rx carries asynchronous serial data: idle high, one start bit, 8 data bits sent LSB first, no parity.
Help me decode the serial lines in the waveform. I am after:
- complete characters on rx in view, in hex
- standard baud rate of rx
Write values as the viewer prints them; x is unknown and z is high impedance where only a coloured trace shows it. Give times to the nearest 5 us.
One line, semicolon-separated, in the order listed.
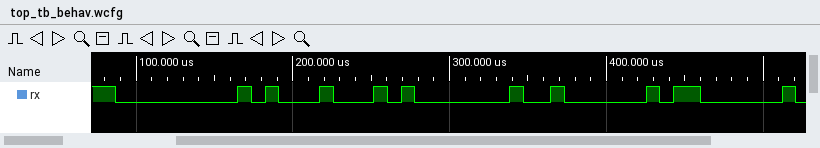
00, 11, 01, 02, 03; 115200 baud
